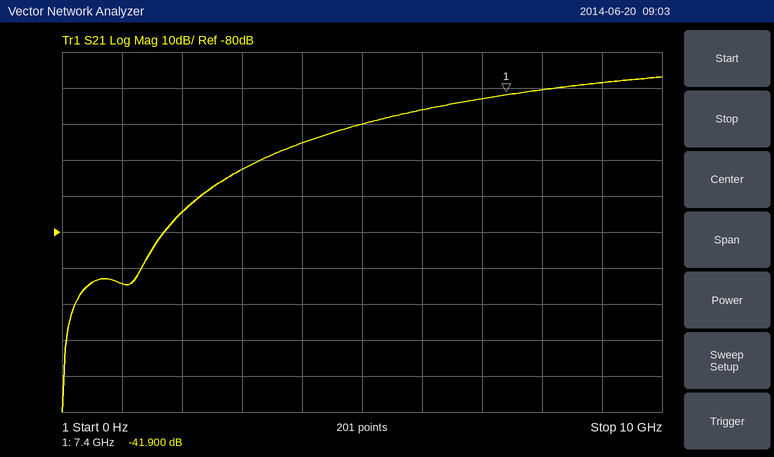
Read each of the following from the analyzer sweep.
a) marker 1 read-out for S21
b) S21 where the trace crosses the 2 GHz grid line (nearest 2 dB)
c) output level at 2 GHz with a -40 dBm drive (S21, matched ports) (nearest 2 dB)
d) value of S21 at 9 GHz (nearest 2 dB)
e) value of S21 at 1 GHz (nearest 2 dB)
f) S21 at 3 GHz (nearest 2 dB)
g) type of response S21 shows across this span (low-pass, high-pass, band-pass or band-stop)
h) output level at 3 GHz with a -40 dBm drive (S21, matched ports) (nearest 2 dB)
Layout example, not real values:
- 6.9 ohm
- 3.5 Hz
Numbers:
- -41.900 dB
- -74 dB
- -114 dBm
- -38 dB
- -94 dB
- -62 dB
- high-pass
- -102 dBm
